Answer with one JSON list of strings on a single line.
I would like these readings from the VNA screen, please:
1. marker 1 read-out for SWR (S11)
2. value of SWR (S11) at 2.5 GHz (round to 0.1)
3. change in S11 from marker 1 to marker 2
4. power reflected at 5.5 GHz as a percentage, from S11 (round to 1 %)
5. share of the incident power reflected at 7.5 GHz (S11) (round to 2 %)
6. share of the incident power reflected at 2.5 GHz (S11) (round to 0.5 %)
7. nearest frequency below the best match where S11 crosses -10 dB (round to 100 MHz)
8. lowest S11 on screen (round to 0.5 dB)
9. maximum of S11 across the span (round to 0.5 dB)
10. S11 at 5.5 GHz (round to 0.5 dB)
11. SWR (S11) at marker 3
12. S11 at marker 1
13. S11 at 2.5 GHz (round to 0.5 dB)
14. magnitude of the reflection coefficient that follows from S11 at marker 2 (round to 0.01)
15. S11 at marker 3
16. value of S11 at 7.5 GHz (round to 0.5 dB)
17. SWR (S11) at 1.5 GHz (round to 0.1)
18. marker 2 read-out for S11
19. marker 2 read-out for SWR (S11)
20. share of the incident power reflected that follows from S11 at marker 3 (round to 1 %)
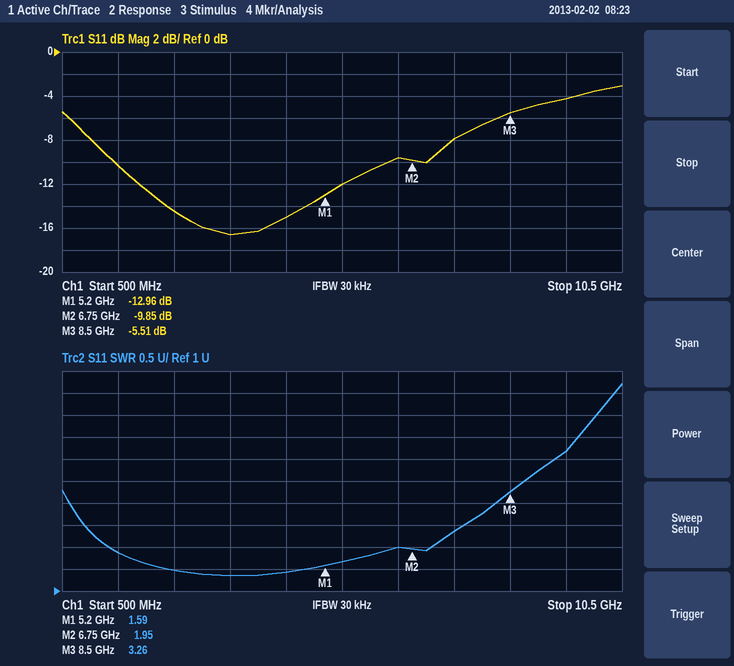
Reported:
["1.59", "1.5", "3.11 dB", "6 %", "16 %", "3.5 %", "1.4 GHz", "-16.5 dB", "-3.0 dB", "-12.0 dB", "3.26", "-12.96 dB", "-14.5 dB", "0.32", "-5.51 dB", "-8.0 dB", "1.9", "-9.85 dB", "1.95", "28 %"]
